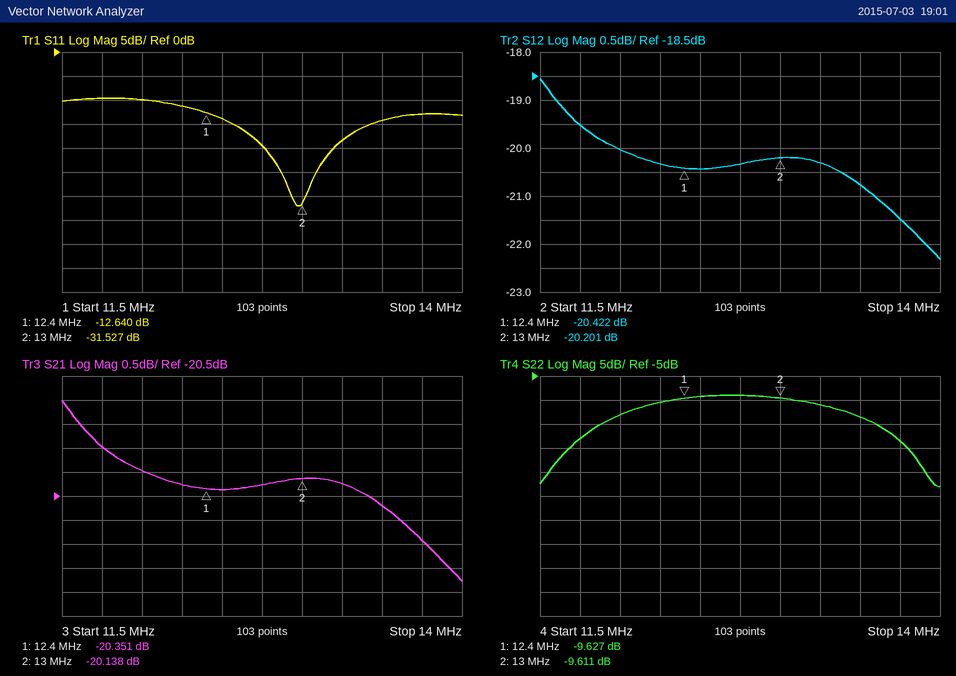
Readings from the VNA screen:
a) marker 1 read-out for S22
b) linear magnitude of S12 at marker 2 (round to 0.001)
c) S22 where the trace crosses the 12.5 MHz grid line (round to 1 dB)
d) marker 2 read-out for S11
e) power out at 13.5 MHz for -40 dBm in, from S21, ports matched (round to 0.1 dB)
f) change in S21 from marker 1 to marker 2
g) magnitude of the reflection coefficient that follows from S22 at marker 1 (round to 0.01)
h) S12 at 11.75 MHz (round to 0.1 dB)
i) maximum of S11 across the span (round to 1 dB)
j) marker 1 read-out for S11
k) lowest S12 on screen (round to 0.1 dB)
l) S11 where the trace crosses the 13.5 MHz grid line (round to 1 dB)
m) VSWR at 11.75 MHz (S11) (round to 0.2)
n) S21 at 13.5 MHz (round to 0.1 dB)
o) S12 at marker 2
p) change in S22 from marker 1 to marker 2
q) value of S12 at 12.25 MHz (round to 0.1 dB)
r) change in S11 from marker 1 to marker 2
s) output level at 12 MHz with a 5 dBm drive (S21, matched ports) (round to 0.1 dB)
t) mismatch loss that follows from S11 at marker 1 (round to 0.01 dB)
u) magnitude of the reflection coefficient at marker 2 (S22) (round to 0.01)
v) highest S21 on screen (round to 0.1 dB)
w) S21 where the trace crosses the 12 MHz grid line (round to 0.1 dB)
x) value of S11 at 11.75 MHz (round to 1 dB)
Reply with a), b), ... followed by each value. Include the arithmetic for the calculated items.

a) -9.627 dB
b) 10^(-20.201/20) ≈ 0.098
c) -9 dB
d) -31.527 dB
e) -40 dBm + (-20.7 dB) = -60.7 dBm
f) -20.138 − (-20.351) = 0.213 dB
g) 10^(-9.627/20) ≈ 0.33
h) -19.5 dB
i) -10 dB
j) -12.640 dB
k) -22.3 dB
l) -14 dB
m) |Γ| = 10^(-10/20) = 0.3162; VSWR = (1 + 0.3162)/(1 − 0.3162) ≈ 1.92, so 2.0 to the nearest 0.2
n) -20.7 dB
o) -20.201 dB
p) -9.611 − (-9.627) = 0.016 dB
q) -20.3 dB
r) -31.527 − (-12.64) = -18.887 dB
s) 5 dBm + (-20.0 dB) = -15.0 dBm
t) −10 log10(1 − 10^(-12.64/10)) ≈ 0.24 dB
u) 10^(-9.611/20) ≈ 0.33
v) -18.5 dB
w) -20.0 dB
x) -10 dB
